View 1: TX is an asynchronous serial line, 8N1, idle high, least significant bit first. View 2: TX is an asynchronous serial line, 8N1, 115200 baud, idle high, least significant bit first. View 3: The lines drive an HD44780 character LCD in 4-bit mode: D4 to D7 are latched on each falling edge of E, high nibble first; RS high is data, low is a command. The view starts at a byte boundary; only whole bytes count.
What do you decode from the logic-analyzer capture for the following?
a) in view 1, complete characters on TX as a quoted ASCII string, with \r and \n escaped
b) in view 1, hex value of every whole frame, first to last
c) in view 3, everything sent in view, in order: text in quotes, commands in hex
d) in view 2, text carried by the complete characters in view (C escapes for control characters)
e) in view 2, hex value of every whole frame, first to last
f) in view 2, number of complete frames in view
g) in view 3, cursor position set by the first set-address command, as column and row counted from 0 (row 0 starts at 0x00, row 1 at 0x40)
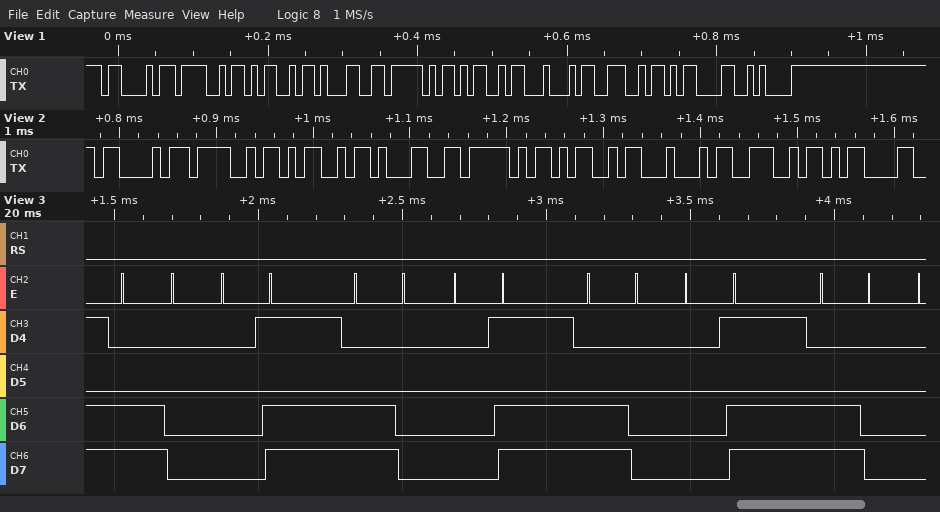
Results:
"COM1_MDN\r\n"
43 4F 4D 31 5F 4D 44 4E 0D 0A
0xC0 0x0D 0xC0 0x0D 0xC0 0x0D 0xC0
"COM1_MDN\r"
43 4F 4D 31 5F 4D 44 4E 0D
9
column 0, row 1
